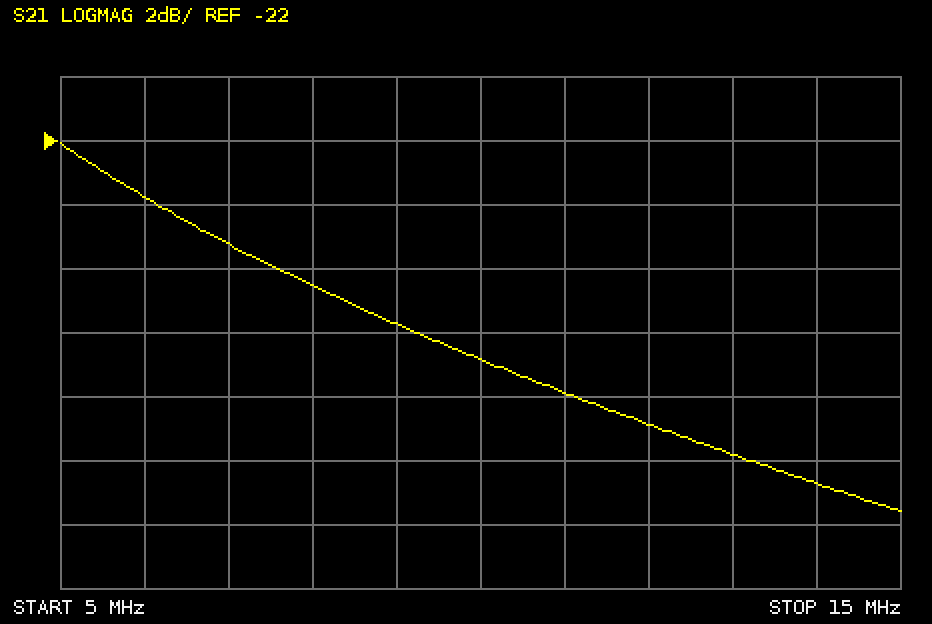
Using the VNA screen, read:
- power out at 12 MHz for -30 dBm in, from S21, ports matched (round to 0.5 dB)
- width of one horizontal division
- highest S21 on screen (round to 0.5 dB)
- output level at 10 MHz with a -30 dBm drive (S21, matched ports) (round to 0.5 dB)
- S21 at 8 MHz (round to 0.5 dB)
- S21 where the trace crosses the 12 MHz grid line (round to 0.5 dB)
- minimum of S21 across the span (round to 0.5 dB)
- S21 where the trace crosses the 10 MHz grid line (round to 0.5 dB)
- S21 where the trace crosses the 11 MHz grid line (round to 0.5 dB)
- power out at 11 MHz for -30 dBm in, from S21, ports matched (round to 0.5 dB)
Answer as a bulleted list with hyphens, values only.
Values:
- -61.0 dBm
- 1 MHz
- -22.0 dB
- -59.0 dBm
- -26.5 dB
- -31.0 dB
- -33.5 dB
- -29.0 dB
- -30.0 dB
- -60.0 dBm
